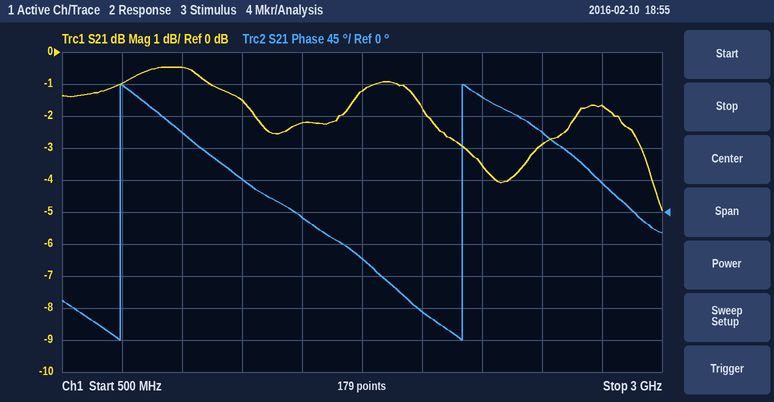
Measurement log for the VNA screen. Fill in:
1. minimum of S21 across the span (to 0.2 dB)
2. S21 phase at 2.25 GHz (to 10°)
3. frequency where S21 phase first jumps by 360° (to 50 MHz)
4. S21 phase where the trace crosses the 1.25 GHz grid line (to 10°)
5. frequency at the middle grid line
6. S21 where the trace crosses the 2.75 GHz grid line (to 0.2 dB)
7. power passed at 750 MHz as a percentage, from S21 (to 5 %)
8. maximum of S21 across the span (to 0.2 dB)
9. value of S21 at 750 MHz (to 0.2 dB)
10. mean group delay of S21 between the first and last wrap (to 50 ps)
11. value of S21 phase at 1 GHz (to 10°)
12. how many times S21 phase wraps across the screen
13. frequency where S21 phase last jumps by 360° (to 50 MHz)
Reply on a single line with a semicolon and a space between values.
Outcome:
-5.0 dB; 160°; 750 MHz; 50°; 1.75 GHz; -1.6 dB; 80 %; -0.4 dB; -1.0 dB; 700 ps; 110°; 2; 2.15 GHz
